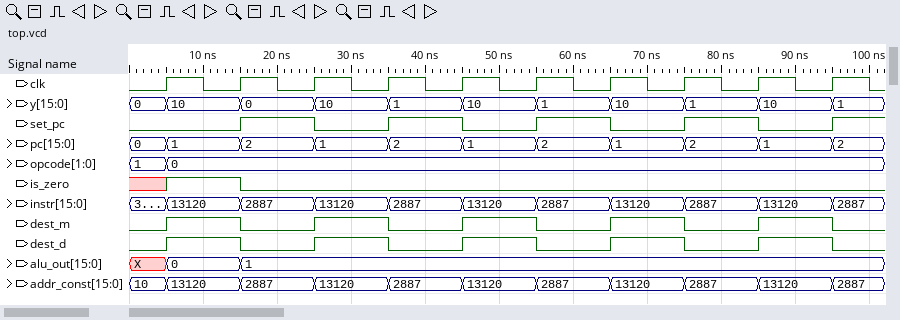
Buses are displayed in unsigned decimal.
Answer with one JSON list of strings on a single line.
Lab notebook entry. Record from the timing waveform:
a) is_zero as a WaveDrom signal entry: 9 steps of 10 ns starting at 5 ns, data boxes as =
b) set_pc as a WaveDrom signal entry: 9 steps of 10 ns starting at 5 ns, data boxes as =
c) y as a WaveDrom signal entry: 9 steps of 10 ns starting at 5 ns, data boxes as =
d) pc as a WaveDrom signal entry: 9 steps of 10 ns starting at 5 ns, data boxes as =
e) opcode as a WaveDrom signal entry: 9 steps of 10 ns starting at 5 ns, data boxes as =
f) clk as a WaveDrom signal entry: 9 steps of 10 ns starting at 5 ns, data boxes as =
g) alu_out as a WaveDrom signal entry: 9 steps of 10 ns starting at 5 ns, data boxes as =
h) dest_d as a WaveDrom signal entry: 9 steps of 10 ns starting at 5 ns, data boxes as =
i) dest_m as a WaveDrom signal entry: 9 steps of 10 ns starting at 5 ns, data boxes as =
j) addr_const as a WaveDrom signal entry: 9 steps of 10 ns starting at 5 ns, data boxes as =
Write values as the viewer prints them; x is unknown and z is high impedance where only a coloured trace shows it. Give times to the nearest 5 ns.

["{name: 'is_zero', wave: '10.......'}", "{name: 'set_pc', wave: '010101010'}", "{name: 'y', wave: '=========', data: '10 0 10 1 10 1 10 1 10'}", "{name: 'pc', wave: '=========', data: '1 2 1 2 1 2 1 2 1'}", "{name: 'opcode', wave: '=........', data: '0'}", "{name: 'clk', wave: 'p........'}", "{name: 'alu_out', wave: '==.......', data: '0 1'}", "{name: 'dest_d', wave: '101010101'}", "{name: 'dest_m', wave: '101010101'}", "{name: 'addr_const', wave: '=========', data: '13120 2887 13120 2887 13120 2887 13120 2887 13120'}"]
